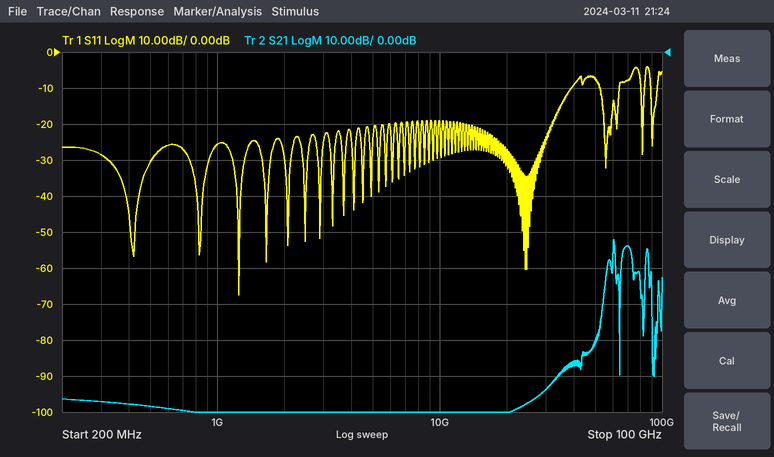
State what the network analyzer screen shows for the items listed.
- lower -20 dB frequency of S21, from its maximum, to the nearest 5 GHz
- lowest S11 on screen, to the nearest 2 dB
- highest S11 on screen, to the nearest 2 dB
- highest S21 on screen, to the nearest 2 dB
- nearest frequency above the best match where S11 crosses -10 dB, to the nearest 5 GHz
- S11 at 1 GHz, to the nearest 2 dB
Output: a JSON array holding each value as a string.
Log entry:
["55 GHz", "-68 dB", "-4 dB", "-52 dB", "40 GHz", "-26 dB"]
